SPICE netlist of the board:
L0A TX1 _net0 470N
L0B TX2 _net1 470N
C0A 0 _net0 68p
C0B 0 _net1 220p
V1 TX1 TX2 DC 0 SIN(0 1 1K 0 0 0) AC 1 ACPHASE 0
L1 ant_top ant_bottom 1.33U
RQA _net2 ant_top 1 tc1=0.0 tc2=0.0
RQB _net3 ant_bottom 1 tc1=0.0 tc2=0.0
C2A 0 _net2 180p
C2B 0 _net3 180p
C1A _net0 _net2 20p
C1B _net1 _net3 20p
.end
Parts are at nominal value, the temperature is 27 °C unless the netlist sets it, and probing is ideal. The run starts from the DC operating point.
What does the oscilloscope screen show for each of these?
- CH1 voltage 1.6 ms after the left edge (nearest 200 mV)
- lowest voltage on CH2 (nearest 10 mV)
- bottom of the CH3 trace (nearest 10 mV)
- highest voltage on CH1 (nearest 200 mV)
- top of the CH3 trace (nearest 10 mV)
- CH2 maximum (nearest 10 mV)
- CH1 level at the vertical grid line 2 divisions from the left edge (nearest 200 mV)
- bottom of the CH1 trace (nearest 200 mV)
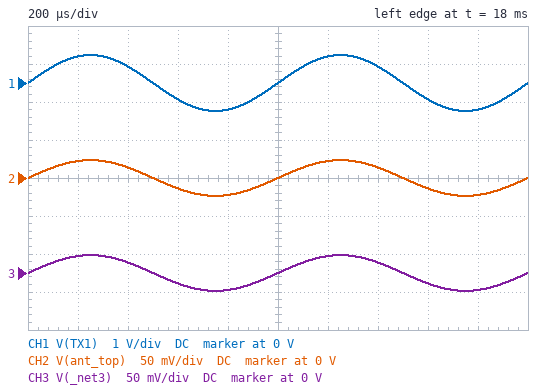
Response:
-400 mV
-20 mV
-20 mV
800 mV
20 mV
20 mV
400 mV
-800 mV
